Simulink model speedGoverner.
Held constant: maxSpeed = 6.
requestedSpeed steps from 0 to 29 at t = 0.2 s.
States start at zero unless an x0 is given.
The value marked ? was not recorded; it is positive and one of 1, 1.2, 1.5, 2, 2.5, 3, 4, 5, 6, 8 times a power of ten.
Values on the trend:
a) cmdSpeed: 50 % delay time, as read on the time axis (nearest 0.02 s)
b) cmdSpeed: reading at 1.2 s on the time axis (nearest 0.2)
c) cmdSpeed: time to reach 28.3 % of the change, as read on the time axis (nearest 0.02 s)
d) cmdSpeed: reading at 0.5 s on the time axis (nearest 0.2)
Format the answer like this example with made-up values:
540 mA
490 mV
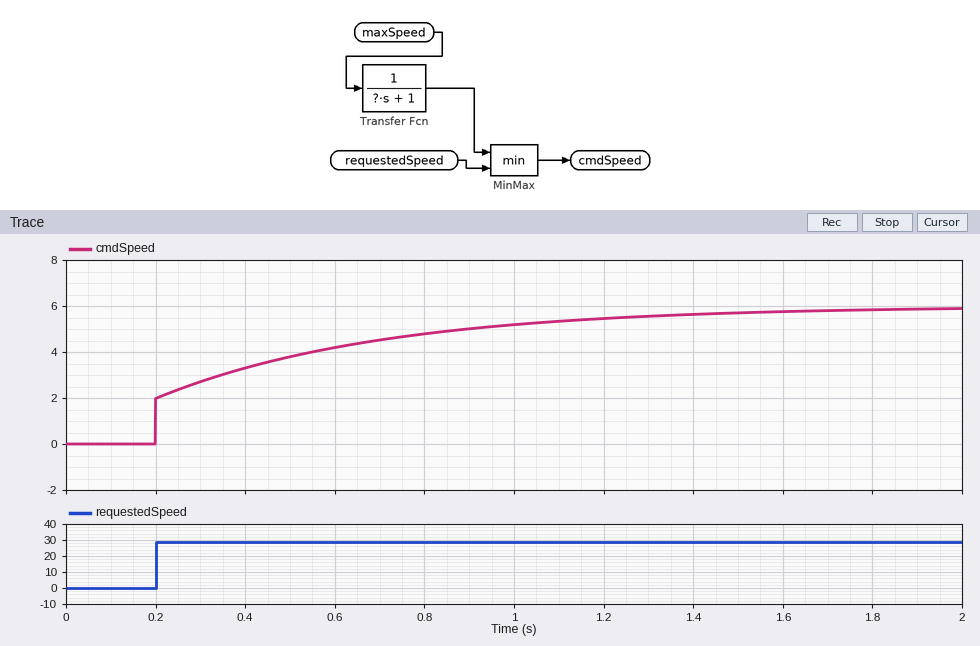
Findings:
0.34 s
5.4
0.20 s
3.8
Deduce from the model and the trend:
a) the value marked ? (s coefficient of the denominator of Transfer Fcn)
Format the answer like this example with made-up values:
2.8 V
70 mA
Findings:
0.5
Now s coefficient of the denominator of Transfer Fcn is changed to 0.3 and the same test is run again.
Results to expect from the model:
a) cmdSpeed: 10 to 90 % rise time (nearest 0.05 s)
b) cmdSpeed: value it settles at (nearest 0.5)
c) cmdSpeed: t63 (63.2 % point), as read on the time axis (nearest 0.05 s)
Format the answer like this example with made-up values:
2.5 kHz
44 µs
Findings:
0.50 s
6.0
0.30 s
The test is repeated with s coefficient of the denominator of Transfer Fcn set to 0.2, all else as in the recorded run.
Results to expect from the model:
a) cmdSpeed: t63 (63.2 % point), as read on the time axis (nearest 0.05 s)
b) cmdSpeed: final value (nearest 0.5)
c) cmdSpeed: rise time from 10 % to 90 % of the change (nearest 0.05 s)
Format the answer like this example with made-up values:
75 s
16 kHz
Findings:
0.20 s
6.0
0.25 s
